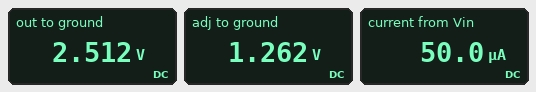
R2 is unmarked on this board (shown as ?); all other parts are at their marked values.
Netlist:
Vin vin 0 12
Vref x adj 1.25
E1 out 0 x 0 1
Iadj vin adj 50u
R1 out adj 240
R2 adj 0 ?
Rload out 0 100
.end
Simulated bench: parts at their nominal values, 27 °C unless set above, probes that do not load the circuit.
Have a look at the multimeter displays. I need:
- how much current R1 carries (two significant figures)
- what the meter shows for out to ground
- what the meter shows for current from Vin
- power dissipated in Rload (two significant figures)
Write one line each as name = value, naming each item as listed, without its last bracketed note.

how much current R1 carries = 5.2 mA
what the meter shows for out to ground = 2.512 V
what the meter shows for current from Vin = 50.0 µA
power dissipated in Rload = 63 mW
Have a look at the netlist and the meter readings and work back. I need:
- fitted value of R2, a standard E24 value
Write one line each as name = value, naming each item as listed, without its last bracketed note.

fitted value of R2, a standard E24 value = 240 Ω
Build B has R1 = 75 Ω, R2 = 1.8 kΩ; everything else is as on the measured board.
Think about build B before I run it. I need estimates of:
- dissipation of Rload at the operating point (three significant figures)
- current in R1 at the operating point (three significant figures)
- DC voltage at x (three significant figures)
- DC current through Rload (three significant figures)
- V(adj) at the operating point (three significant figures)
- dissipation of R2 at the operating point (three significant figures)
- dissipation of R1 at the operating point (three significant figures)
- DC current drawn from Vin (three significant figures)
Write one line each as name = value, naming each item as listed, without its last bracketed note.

dissipation of Rload at the operating point = 9.82 W
current in R1 at the operating point = 16.7 mA
DC voltage at x = 31.3 V
DC current through Rload = 313 mA
V(adj) at the operating point = 30.1 V
dissipation of R2 at the operating point = 503 mW
dissipation of R1 at the operating point = 20.8 mW
DC current drawn from Vin = 50.0 µA
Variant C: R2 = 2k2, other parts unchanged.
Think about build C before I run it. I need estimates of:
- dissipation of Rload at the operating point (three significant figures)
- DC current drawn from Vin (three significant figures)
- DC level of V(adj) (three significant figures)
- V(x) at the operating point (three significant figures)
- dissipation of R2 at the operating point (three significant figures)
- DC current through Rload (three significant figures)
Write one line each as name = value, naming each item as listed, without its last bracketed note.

dissipation of Rload at the operating point = 1.64 W
DC current drawn from Vin = 50.0 µA
DC level of V(adj) = 11.6 V
V(x) at the operating point = 12.8 V
dissipation of R2 at the operating point = 60.8 mW
DC current through Rload = 128 mA
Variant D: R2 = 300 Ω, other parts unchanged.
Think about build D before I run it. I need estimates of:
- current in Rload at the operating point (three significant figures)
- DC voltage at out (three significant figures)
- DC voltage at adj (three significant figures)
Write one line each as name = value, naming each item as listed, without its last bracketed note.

current in Rload at the operating point = 28.3 mA
DC voltage at out = 2.83 V
DC voltage at adj = 1.58 V
